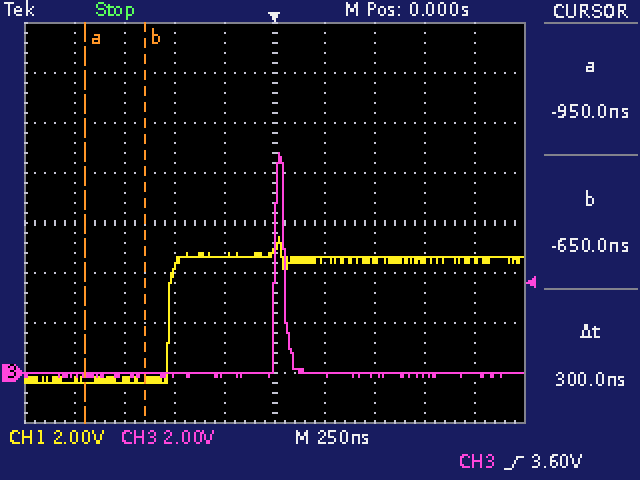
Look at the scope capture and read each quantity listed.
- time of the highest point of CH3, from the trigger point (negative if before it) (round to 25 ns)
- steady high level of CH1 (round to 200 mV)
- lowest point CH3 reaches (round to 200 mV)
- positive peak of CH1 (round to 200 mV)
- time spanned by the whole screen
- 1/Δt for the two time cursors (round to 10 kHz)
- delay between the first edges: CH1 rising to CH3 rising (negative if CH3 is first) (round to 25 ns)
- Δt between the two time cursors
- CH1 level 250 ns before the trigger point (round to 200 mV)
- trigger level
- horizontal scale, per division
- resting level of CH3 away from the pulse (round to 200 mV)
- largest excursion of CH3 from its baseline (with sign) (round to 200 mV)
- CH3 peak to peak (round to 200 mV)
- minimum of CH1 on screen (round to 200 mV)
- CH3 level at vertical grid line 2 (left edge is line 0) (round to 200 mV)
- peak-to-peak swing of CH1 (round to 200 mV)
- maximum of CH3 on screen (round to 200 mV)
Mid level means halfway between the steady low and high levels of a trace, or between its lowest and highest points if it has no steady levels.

+25 ns
4.6 V
-200 mV
5.4 V
2.5 µs
3.33 MHz
+525 ns
300 ns
4.6 V
3.60 V
250 ns
0.0 V
+8.8 V
9.0 V
-400 mV
0.0 V
5.8 V
8.8 V
